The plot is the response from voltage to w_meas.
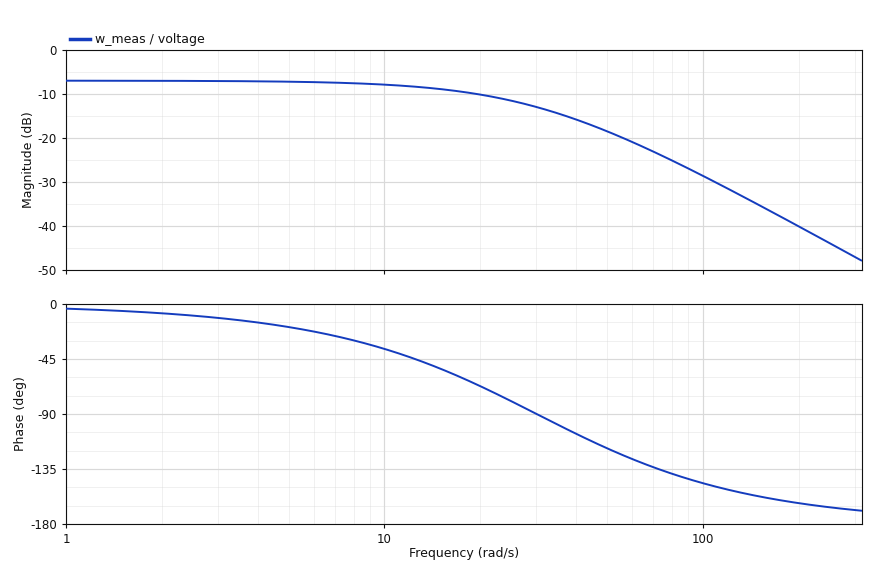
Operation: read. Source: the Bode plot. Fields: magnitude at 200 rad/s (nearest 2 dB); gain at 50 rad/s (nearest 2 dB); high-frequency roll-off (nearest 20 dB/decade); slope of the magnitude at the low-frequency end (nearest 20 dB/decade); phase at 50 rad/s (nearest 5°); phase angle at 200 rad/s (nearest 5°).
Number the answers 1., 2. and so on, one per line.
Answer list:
1. -40 dB
2. -18 dB
3. -40 dB/decade
4. 0 dB/decade
5. -120°
6. -165°
